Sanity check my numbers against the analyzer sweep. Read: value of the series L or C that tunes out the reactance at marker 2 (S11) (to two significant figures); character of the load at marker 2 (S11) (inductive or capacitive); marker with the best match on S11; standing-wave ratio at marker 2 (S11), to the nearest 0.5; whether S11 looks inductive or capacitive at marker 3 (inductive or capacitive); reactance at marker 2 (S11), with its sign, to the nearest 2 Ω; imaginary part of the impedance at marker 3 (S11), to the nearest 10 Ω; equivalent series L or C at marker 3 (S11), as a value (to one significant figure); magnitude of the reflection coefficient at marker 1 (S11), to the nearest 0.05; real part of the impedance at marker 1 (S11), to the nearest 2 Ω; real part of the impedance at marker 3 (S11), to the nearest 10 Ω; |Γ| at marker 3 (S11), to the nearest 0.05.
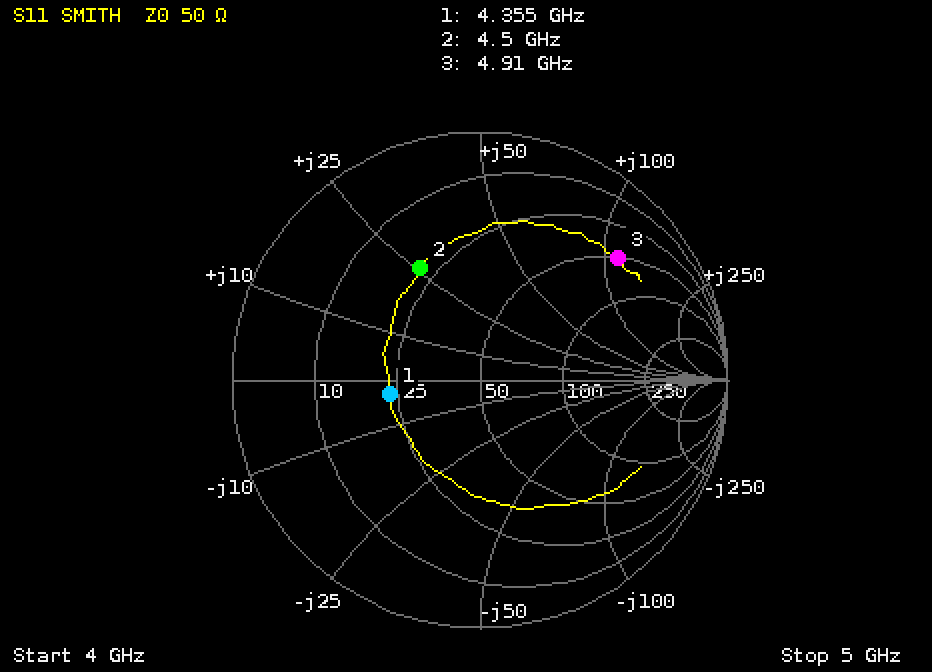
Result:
1.4 pF
inductive
marker 1
3.0
inductive
+26 Ω
+110 Ω
4 nH
0.35
24 Ω
50 Ω
0.75
